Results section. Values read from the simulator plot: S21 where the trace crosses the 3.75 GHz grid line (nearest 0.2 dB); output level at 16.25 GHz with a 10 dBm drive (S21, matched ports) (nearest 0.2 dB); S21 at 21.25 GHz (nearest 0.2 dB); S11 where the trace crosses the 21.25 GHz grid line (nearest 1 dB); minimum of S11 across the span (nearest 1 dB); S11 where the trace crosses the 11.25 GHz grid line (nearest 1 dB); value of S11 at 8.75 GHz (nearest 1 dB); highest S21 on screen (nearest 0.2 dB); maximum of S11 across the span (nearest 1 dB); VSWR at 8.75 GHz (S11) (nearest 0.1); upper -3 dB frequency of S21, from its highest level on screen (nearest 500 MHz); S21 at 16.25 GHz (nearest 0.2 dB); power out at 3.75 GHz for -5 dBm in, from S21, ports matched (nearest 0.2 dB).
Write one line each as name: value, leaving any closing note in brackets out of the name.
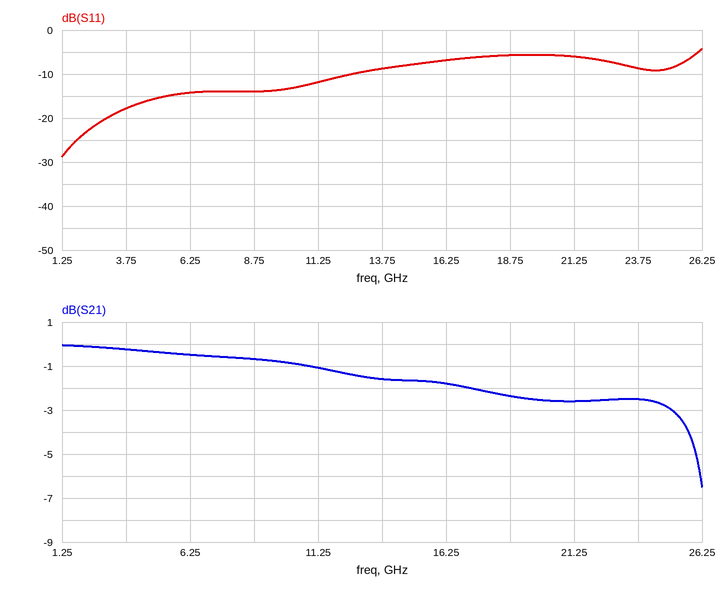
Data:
S21 where the trace crosses the 3.75 GHz grid line: -0.2 dB
output level at 16.25 GHz with a 10 dBm drive (S21, matched ports): 8.2 dBm
S21 at 21.25 GHz: -2.6 dB
S11 where the trace crosses the 21.25 GHz grid line: -6 dB
minimum of S11 across the span: -29 dB
S11 where the trace crosses the 11.25 GHz grid line: -12 dB
value of S11 at 8.75 GHz: -14 dB
highest S21 on screen: 0.0 dB
maximum of S11 across the span: -4 dB
VSWR at 8.75 GHz (S11): 1.5
upper -3 dB frequency of S21, from its highest level on screen: 25.0 GHz
S21 at 16.25 GHz: -1.8 dB
power out at 3.75 GHz for -5 dBm in, from S21, ports matched: -5.2 dBm
